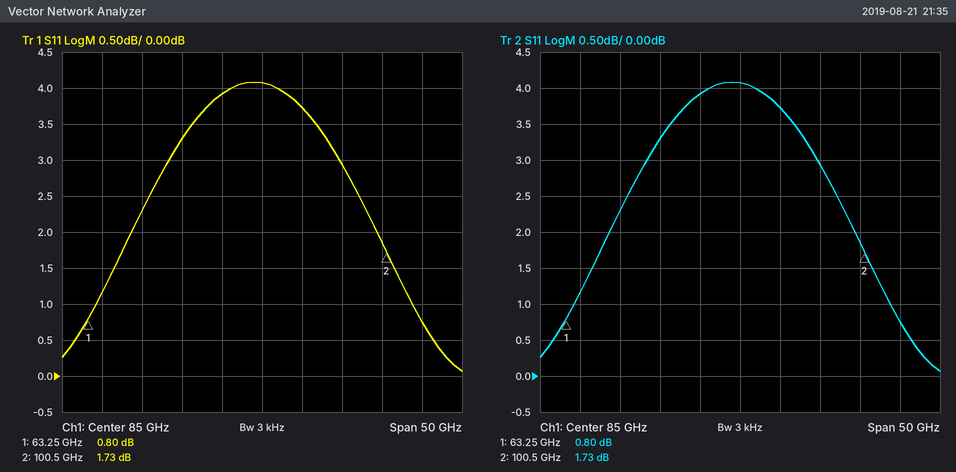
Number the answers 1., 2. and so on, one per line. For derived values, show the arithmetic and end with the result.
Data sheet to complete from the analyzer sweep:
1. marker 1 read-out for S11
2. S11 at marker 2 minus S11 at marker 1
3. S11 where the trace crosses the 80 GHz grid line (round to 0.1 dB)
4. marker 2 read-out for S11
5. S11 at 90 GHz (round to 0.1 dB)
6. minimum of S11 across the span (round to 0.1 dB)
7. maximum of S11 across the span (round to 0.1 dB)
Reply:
1. 0.80 dB
2. 1.73 − (0.8) = 0.93 dB
3. 3.9 dB
4. 1.73 dB
5. 3.7 dB
6. 0.1 dB
7. 4.1 dB
